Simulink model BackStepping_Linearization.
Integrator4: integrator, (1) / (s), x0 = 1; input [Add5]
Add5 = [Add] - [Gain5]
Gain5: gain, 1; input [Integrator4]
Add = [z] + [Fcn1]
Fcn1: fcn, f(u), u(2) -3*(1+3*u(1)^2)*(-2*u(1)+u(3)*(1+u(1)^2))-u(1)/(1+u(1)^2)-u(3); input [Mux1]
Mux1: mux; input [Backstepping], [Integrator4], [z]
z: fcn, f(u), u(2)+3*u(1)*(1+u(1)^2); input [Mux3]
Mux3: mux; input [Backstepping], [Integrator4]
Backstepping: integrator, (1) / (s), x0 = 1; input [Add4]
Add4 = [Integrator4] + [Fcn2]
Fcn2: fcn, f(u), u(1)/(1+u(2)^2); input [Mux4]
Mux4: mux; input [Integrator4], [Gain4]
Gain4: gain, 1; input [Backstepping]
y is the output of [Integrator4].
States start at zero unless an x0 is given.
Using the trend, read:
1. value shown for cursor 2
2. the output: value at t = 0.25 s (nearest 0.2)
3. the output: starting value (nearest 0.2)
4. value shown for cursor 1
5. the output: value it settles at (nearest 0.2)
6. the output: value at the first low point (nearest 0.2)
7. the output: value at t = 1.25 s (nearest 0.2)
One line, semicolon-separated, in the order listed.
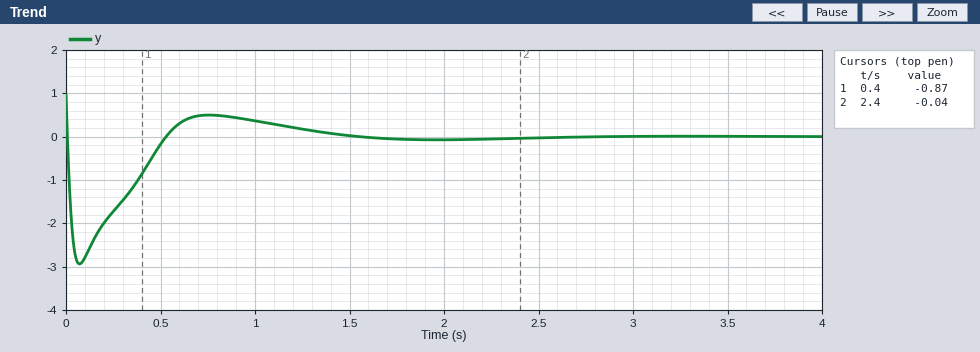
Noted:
-0.04; -1.8; 1.0; -0.87; 0.0; -3.0; 0.2
